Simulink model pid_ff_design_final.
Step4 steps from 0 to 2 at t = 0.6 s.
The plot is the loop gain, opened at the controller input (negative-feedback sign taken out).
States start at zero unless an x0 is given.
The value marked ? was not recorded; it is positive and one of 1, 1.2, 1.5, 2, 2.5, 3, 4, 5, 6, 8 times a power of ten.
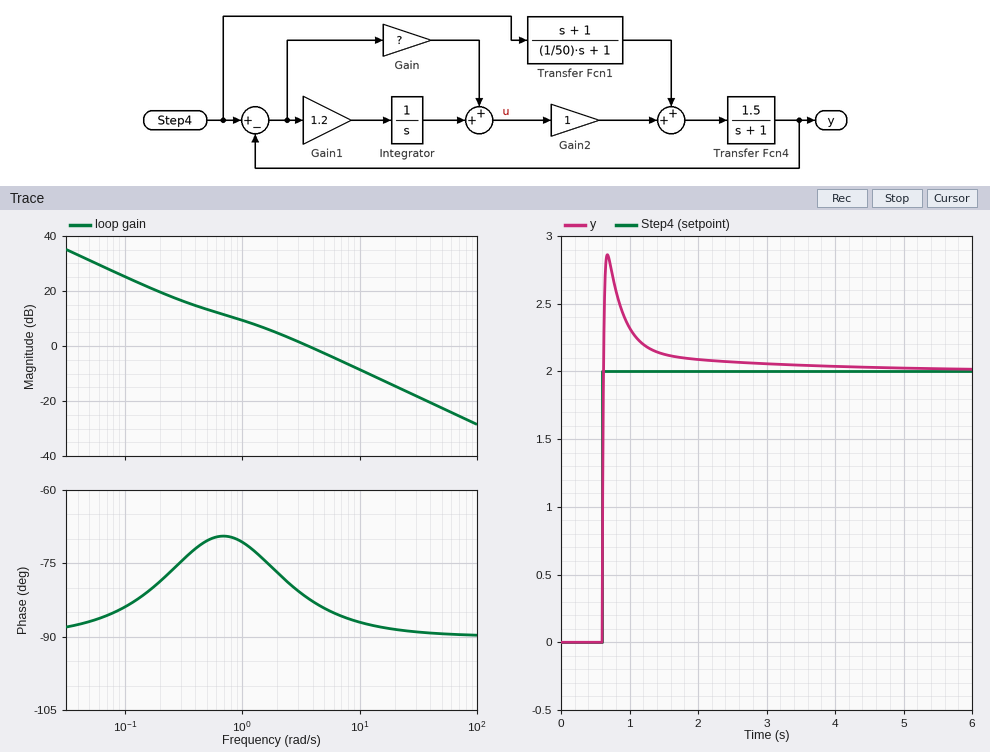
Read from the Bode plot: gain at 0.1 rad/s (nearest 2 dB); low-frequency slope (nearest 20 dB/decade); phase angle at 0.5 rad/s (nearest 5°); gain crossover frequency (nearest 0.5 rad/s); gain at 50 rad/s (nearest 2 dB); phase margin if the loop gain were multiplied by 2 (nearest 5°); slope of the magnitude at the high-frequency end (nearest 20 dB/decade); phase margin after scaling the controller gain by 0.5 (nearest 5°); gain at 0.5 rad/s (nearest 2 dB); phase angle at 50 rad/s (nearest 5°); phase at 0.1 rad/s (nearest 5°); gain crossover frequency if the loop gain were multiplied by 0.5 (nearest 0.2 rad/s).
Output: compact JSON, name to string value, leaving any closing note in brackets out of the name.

{"gain at 0.1 rad/s": "26 dB", "low-frequency slope": "-20 dB/decade", "phase angle at 0.5 rad/s": "-70°", "gain crossover frequency": "3.5 rad/s", "gain at 50 rad/s": "-22 dB", "phase margin if the loop gain were multiplied by 2": "95°", "slope of the magnitude at the high-frequency end": "-20 dB/decade", "phase margin after scaling the controller gain by 0.5": "105°", "gain at 0.5 rad/s": "14 dB", "phase angle at 50 rad/s": "-90°", "phase at 0.1 rad/s": "-85°", "gain crossover frequency if the loop gain were multiplied by 0.5": "1.6 rad/s"}
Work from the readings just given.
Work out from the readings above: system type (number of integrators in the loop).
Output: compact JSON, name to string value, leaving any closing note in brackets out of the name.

{"system type": "1"}
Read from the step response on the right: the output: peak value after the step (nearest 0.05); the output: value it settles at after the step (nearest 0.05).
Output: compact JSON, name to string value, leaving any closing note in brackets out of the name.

{"the output: peak value after the step": "2.85", "the output: value it settles at after the step": "2.00"}
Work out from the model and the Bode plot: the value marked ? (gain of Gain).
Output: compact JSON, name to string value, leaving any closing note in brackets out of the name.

{"the value marked ?": "2.5"}
